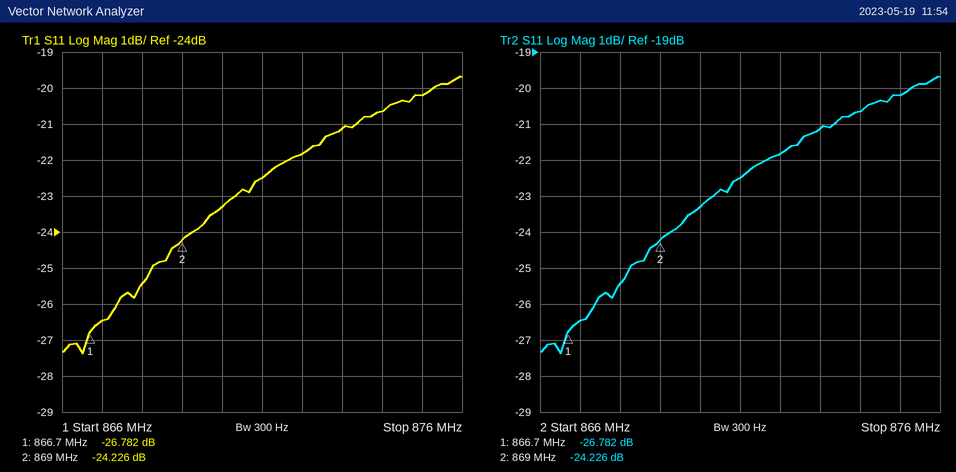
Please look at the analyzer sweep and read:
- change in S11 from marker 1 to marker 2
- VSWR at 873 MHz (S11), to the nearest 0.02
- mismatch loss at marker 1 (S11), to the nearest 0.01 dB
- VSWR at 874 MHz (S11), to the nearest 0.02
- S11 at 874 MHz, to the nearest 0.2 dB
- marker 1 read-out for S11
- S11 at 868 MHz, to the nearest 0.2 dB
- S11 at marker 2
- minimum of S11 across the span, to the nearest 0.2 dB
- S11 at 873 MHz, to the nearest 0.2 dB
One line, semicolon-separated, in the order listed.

2.556 dB; 1.20; 0.01 dB; 1.20; -20.6 dB; -26.782 dB; -25.4 dB; -24.226 dB; -27.4 dB; -21.2 dB
